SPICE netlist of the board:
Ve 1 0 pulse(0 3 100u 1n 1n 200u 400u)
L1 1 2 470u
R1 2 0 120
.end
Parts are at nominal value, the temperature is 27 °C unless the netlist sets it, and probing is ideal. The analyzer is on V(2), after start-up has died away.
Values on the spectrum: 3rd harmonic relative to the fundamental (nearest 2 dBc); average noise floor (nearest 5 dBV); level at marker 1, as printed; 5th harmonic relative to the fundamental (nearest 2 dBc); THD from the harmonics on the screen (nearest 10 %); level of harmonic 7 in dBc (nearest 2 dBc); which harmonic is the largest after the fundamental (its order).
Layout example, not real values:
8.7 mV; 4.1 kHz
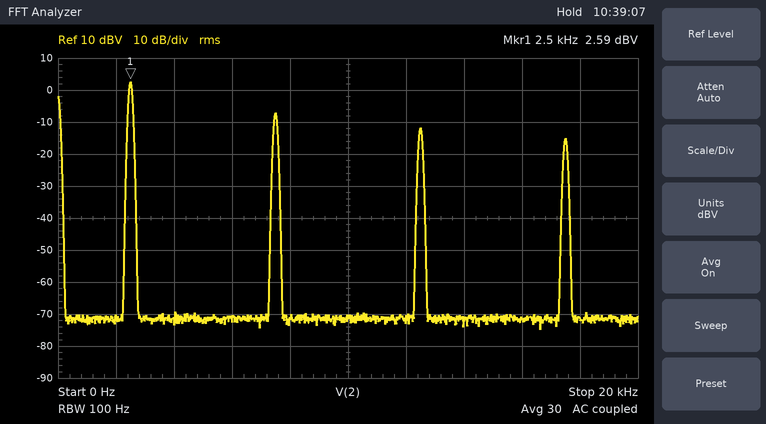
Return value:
-10 dBc; -70 dBV; 2.59 dBV; -14 dBc; 40 %; -18 dBc; 3
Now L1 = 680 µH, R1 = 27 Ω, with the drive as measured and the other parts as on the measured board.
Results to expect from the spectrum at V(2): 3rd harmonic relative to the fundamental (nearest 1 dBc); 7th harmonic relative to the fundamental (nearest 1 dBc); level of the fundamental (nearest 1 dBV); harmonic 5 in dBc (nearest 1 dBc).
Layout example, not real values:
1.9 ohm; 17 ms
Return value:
-13 dBc; -26 dBc; 2 dBV; -20 dBc
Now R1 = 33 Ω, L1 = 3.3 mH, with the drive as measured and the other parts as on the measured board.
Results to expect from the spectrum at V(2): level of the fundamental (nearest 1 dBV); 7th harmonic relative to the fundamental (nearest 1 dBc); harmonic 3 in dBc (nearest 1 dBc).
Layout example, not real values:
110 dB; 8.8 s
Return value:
-3 dBV; -32 dBc; -18 dBc
